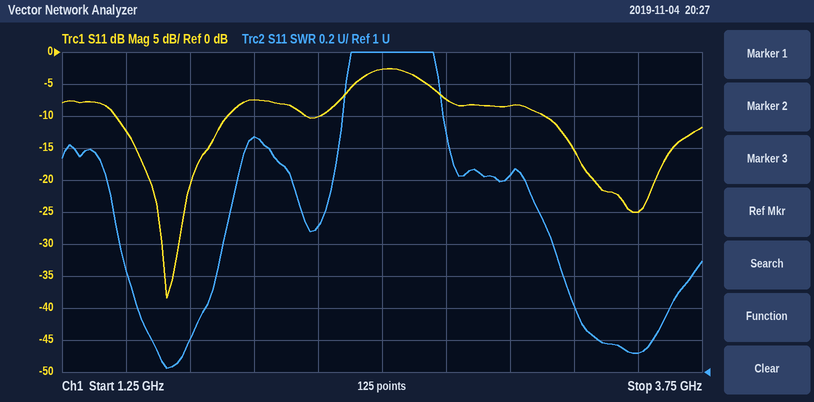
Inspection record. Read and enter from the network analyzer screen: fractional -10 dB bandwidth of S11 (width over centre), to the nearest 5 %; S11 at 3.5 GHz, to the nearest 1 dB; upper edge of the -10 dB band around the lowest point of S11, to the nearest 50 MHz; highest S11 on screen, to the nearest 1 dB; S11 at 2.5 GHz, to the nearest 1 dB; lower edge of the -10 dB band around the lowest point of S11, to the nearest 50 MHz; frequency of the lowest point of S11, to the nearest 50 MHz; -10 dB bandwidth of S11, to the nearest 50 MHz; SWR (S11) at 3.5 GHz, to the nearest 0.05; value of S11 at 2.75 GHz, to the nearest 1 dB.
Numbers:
25 %
-25 dB
1.90 GHz
-3 dB
-3 dB
1.45 GHz
1.65 GHz
450 MHz
1.10
-7 dB
